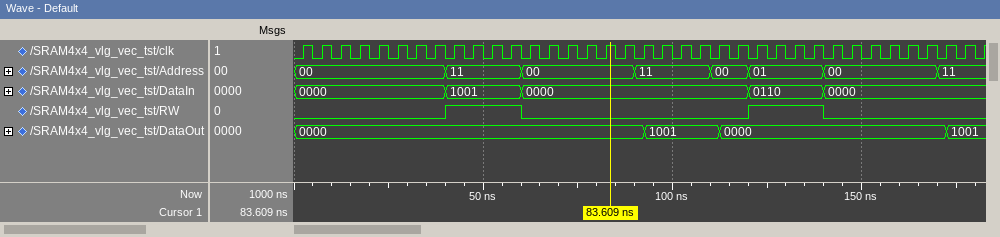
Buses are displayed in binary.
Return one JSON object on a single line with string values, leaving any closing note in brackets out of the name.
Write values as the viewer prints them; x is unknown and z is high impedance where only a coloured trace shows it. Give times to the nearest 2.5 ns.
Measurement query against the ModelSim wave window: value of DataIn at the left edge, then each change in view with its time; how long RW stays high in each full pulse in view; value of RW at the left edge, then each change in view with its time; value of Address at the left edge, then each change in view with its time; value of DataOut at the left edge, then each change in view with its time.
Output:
{"value of DataIn at the left edge, then each change in view with its time": "0000, 1001 at 40 ns, 0000 at 60 ns, 0110 at 120 ns, 0000 at 140 ns", "how long RW stays high in each full pulse in view": "20 ns, 20 ns", "value of RW at the left edge, then each change in view with its time": "0, 1 at 40 ns, 0 at 60 ns, 1 at 120 ns, 0 at 140 ns", "value of Address at the left edge, then each change in view with its time": "00, 11 at 40 ns, 00 at 60 ns, 11 at 90 ns, 00 at 110 ns, 01 at 120 ns, 00 at 140 ns, 11 at 170 ns", "value of DataOut at the left edge, then each change in view with its time": "0000, 1001 at 92.5 ns, 0000 at 112.5 ns, 1001 at 172.5 ns"}
